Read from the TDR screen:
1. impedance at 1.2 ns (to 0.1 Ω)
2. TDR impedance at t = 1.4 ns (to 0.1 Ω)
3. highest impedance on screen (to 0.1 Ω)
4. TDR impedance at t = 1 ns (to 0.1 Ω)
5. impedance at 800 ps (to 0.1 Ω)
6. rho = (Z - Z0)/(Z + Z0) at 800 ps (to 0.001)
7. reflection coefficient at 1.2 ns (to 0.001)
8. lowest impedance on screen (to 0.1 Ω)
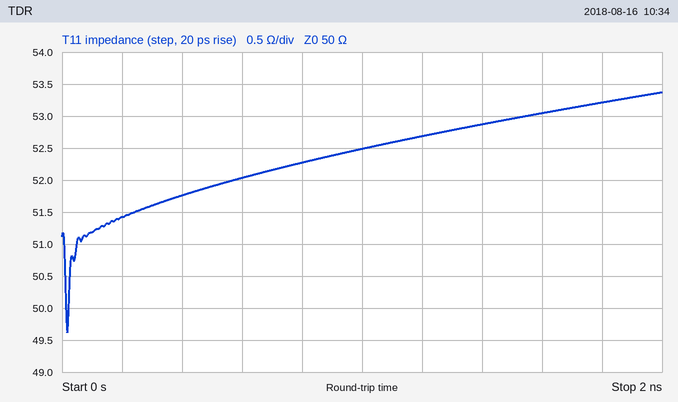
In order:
52.7 Ω
52.9 Ω
53.4 Ω
52.5 Ω
52.3 Ω
+0.022
+0.026
49.6 Ω
